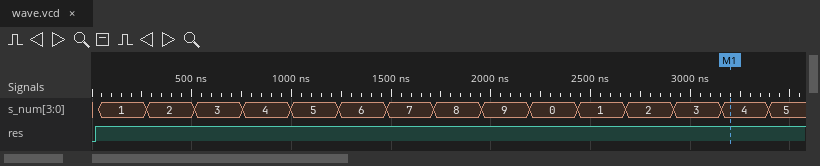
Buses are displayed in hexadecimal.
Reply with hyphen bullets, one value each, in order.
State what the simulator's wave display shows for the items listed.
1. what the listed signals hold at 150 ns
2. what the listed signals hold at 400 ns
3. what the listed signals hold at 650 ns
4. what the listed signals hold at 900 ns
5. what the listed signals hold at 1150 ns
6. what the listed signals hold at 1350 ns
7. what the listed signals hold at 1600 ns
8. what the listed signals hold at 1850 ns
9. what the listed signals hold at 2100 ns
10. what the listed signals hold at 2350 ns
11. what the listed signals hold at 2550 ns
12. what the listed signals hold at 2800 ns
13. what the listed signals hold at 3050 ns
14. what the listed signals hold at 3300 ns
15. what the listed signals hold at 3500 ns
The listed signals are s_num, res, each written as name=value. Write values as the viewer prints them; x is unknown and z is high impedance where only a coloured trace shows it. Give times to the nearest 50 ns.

- s_num=1, res=1
- s_num=2, res=1
- s_num=3, res=1
- s_num=4, res=1
- s_num=5, res=1
- s_num=6, res=1
- s_num=7, res=1
- s_num=8, res=1
- s_num=9, res=1
- s_num=0, res=1
- s_num=1, res=1
- s_num=2, res=1
- s_num=3, res=1
- s_num=4, res=1
- s_num=5, res=1
